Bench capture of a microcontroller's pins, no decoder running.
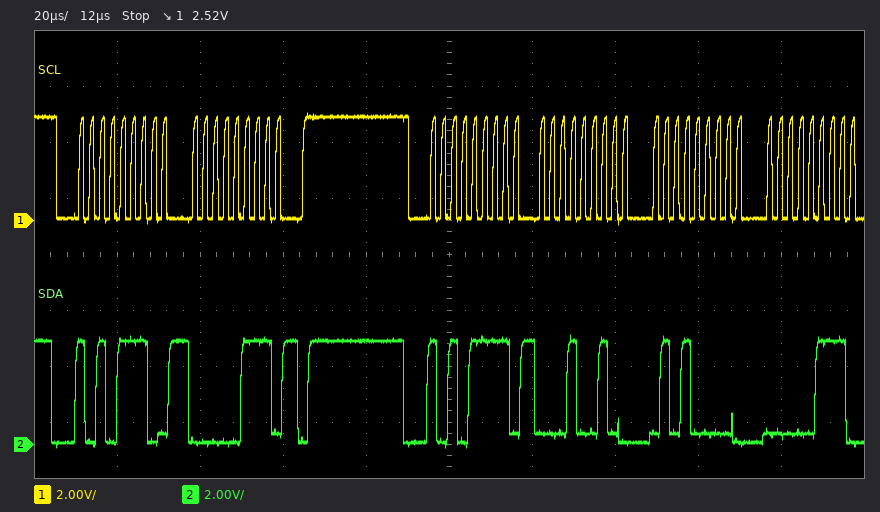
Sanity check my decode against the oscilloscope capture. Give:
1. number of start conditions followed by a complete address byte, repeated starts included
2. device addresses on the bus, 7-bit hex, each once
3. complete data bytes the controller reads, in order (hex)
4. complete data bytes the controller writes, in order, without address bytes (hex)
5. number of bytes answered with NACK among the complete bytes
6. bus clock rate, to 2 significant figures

2
0x57
12 50 07
07
0
400 kHz
